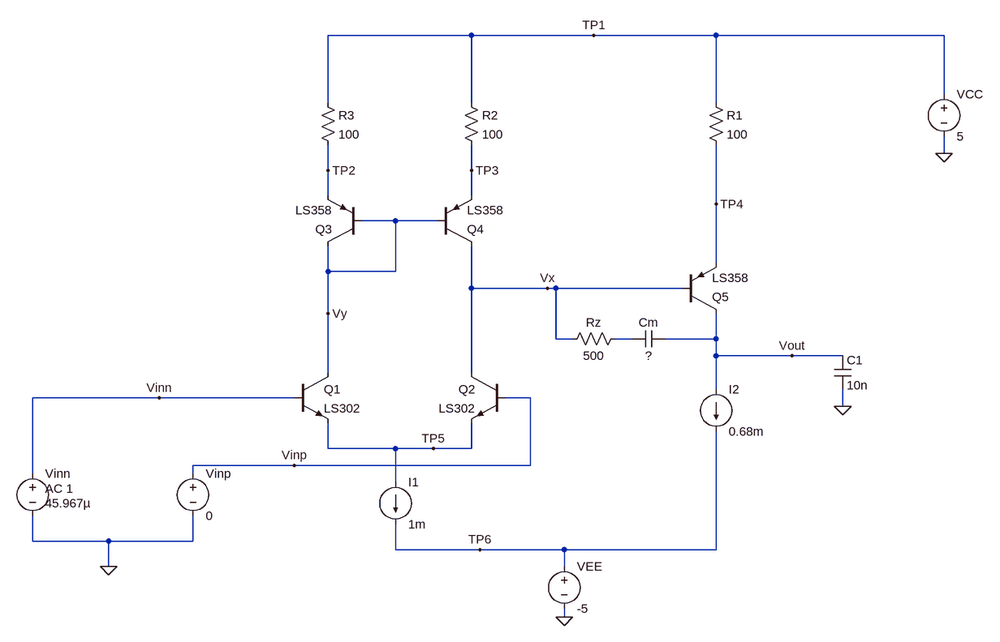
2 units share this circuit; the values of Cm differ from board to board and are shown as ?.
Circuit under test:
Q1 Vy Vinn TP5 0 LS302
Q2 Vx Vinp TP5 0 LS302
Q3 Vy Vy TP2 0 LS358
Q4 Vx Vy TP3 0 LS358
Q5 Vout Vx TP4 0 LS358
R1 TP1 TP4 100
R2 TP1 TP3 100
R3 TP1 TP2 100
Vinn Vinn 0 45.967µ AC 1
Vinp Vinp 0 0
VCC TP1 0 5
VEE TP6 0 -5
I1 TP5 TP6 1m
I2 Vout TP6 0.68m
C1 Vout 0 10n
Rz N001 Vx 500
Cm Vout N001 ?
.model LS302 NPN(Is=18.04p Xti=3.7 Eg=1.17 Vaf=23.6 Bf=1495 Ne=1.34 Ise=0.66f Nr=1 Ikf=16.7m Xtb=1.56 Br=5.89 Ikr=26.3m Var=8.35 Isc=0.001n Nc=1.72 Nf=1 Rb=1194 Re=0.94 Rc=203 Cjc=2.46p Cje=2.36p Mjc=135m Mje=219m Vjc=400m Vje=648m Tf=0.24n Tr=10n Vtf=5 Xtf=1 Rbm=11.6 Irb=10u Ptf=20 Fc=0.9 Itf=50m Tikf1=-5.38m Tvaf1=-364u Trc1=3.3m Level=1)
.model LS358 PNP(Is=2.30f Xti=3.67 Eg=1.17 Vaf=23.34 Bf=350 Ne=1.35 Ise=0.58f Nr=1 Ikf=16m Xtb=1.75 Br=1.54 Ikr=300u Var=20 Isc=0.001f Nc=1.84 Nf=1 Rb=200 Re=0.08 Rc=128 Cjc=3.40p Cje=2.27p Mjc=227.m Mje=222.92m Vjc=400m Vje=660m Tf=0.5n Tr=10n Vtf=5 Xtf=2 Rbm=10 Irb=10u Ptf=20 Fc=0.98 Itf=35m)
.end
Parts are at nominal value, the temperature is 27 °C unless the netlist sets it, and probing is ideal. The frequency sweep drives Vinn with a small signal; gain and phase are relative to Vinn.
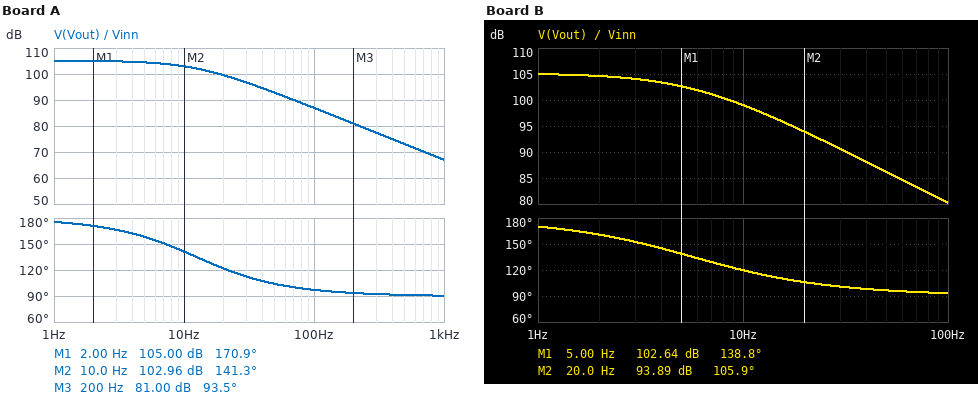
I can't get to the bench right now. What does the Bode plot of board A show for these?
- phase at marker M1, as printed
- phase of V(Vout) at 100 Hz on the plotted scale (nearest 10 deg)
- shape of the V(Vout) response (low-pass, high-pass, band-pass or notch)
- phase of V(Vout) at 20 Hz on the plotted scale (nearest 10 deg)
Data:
170.9 deg
100 deg
low-pass
120 deg
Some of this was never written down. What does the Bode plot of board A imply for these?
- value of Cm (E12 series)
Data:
1.2 nF
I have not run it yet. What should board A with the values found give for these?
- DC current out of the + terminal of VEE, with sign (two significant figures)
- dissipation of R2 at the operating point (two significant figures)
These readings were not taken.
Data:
-1.7 mA
25 µW
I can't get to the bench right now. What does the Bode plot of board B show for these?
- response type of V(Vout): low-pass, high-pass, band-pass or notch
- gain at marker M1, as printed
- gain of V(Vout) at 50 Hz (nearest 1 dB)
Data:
low-pass
102.64 dB
86 dB
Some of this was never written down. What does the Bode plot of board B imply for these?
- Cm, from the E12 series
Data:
2.7 nF
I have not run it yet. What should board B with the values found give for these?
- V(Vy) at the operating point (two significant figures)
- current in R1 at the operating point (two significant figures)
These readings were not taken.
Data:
4.3 V
680 µA
